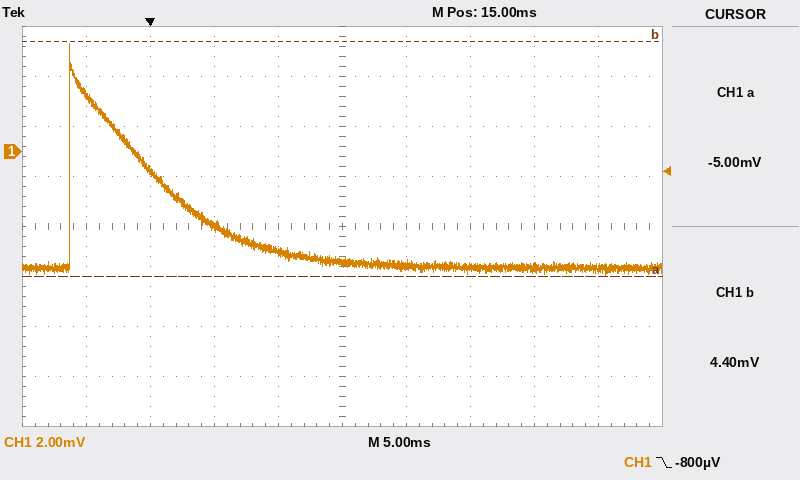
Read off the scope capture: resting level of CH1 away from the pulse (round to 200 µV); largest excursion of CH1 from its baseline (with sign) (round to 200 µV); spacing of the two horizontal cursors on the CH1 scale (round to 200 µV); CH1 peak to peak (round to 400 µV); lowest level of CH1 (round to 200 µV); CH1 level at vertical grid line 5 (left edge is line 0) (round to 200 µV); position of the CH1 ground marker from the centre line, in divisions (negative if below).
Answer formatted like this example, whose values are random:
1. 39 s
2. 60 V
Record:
1. -4.6 mV
2. +9.0 mV
3. 9.4 mV
4. 9.2 mV
5. -5.0 mV
6. -4.4 mV
7. +1.5 div
